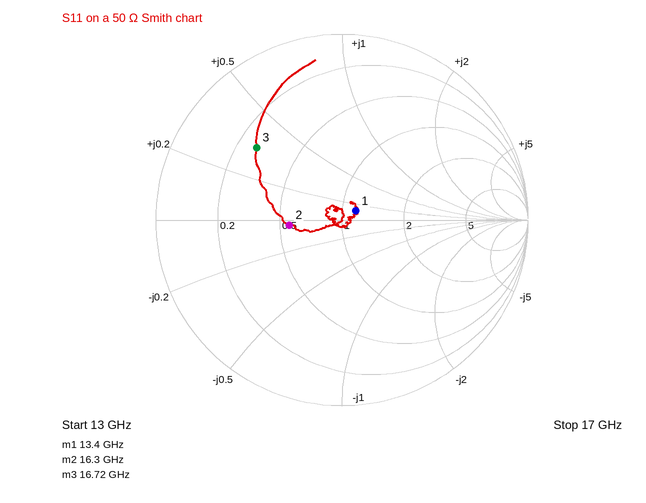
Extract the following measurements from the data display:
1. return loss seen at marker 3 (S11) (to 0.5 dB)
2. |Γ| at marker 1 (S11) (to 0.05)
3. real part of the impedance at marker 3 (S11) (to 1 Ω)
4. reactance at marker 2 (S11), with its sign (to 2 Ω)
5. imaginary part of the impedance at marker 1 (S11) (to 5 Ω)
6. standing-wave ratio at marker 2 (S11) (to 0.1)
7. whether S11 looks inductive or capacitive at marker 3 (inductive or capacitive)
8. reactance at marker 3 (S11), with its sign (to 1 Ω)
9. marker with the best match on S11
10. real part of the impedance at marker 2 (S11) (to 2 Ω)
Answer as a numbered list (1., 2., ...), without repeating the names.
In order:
1. 4.5 dB
2. 0.10
3. 14 Ω
4. -2 Ω
5. +5 Ω
6. 1.8
7. inductive
8. +17 Ω
9. marker 1
10. 28 Ω
